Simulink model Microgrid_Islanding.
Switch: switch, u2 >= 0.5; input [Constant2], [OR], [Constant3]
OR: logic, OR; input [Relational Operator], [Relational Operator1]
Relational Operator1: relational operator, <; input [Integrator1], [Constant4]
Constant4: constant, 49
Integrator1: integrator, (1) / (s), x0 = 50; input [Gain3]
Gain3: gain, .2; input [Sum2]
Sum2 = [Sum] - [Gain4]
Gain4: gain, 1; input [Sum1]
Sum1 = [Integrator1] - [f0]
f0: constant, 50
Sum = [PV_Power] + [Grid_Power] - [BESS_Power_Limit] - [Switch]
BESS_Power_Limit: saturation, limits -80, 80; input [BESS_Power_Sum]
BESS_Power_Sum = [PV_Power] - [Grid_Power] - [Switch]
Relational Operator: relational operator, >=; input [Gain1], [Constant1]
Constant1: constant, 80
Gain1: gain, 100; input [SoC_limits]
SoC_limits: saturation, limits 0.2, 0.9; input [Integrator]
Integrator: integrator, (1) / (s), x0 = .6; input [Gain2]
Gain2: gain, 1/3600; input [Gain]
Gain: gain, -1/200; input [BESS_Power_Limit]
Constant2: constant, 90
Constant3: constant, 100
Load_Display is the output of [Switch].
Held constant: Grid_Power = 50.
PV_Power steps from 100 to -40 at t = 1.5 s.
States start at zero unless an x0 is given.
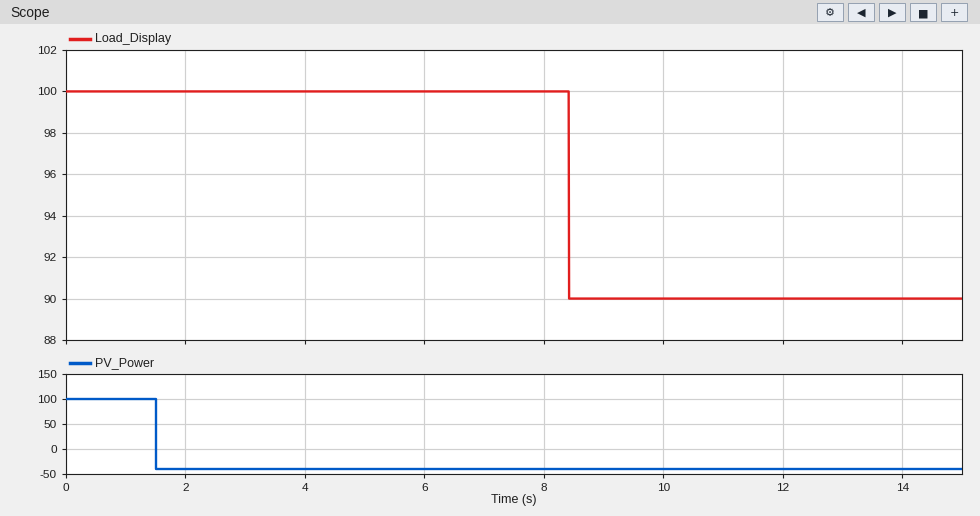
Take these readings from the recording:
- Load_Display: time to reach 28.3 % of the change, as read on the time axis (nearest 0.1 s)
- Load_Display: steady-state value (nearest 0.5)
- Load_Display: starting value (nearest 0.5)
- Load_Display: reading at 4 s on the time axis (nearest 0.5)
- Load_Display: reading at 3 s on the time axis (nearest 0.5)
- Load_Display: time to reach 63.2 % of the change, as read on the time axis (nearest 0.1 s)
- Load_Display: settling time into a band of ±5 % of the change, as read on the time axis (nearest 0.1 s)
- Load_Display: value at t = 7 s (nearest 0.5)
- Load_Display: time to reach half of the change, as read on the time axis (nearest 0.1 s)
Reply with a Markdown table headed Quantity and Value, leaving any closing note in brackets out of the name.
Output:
| Quantity | Value |
|---|---|
| Load_Display: time to reach 28.3 % of the change, as read on the time axis | 8.4 s |
| Load_Display: steady-state value | 90.0 |
| Load_Display: starting value | 100.0 |
| Load_Display: reading at 4 s on the time axis | 100.0 |
| Load_Display: reading at 3 s on the time axis | 100.0 |
| Load_Display: time to reach 63.2 % of the change, as read on the time axis | 8.4 s |
| Load_Display: settling time into a band of ±5 % of the change, as read on the time axis | 8.4 s |
| Load_Display: value at t = 7 s | 100.0 |
| Load_Display: time to reach half of the change, as read on the time axis | 8.4 s |
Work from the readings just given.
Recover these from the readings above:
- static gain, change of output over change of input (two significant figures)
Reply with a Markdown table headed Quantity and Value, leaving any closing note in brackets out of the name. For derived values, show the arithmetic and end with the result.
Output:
| Quantity | Value |
|---|---|
| static gain, change of output over change of input | (90 - 100) / (-40 - 100) = 0.071 |
